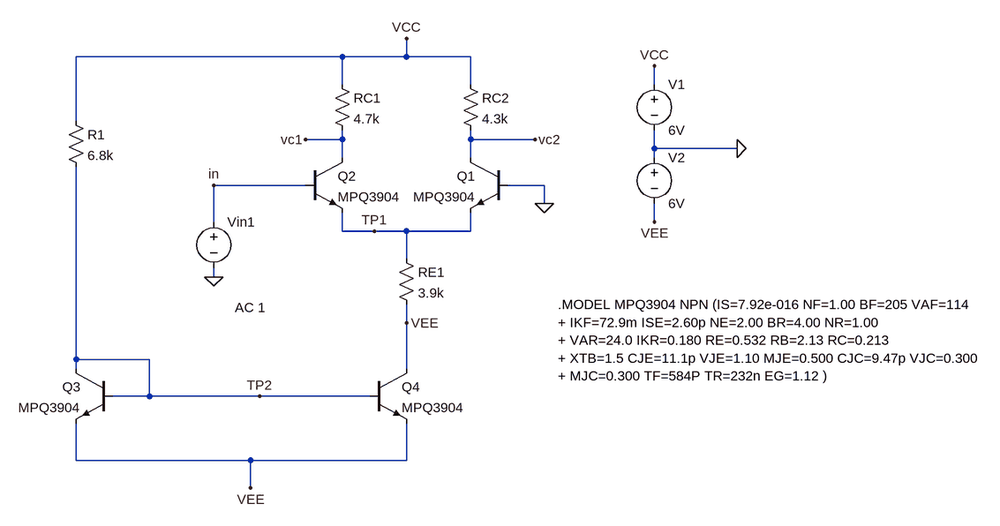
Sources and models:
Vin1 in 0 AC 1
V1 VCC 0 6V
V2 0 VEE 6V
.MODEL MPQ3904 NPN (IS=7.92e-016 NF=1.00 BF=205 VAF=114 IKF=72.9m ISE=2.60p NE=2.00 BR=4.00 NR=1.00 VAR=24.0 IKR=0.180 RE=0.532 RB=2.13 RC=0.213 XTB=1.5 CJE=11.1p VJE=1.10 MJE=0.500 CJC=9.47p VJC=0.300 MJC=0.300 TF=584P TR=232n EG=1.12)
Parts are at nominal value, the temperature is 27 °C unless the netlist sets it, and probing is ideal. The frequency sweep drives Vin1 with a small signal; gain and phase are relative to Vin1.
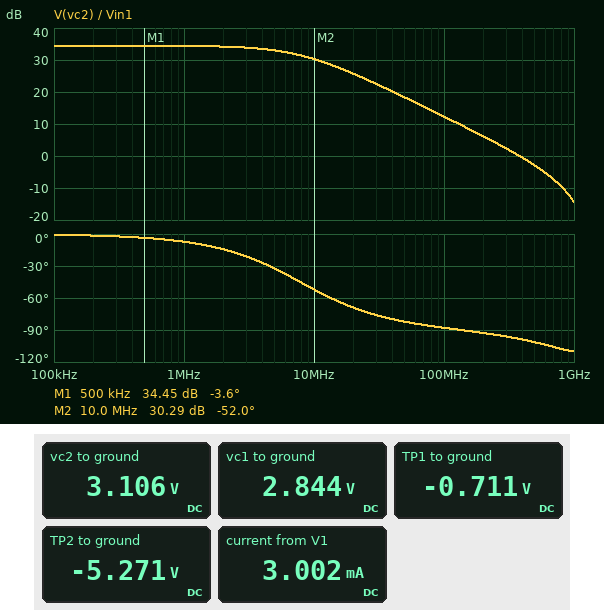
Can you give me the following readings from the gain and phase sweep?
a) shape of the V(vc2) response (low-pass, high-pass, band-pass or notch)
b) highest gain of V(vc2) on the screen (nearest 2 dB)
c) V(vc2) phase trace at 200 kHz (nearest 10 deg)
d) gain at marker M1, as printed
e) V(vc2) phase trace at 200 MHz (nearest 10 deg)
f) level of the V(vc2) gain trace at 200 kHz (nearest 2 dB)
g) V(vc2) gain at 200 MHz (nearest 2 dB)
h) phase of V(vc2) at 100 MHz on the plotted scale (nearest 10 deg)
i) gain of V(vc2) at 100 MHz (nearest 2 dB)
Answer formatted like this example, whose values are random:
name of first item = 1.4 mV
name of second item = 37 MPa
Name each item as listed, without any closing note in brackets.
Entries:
shape of the V(vc2) response = low-pass
highest gain of V(vc2) on the screen = 34 dB
V(vc2) phase trace at 200 kHz = 0 deg
gain at marker M1, as printed = 34.45 dB
V(vc2) phase trace at 200 MHz = -90 deg
level of the V(vc2) gain trace at 200 kHz = 34 dB
V(vc2) gain at 200 MHz = 6 dB
phase of V(vc2) at 100 MHz on the plotted scale = -90 deg
gain of V(vc2) at 100 MHz = 12 dB
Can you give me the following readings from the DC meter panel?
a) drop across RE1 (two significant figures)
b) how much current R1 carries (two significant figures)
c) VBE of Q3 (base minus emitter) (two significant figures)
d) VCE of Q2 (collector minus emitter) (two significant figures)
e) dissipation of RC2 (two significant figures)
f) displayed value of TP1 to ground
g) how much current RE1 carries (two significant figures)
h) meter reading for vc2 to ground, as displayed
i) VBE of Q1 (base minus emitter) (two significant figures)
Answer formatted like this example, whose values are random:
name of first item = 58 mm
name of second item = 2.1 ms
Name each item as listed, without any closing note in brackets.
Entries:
drop across RE1 = 5.3 V
how much current R1 carries = 1.7 mA
VBE of Q3 (base minus emitter) = 730 mV
VCE of Q2 (collector minus emitter) = 3.6 V
dissipation of RC2 = 1.9 mW
displayed value of TP1 to ground = -0.711 V
how much current RE1 carries = 1.4 mA
meter reading for vc2 to ground, as displayed = 3.106 V
VBE of Q1 (base minus emitter) = 710 mV
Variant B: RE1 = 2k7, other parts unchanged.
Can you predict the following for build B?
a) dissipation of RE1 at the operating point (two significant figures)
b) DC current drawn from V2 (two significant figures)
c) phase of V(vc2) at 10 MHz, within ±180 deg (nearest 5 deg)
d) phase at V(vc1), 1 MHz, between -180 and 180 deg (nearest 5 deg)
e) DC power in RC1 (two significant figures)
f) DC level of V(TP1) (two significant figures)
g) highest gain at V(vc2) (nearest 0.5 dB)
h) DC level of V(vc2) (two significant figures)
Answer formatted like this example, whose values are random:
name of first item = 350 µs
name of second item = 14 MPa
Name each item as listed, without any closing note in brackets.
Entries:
dissipation of RE1 at the operating point = 10 mW
DC current drawn from V2 = 3.6 mA
phase of V(vc2) at 10 MHz, within ±180 deg = -55 deg
phase at V(vc1), 1 MHz, between -180 and 180 deg = 170 deg
DC power in RC1 = 4.4 mW
DC level of V(TP1) = -720 mV
highest gain at V(vc2) = 37.5 dB
DC level of V(vc2) = 1.8 V
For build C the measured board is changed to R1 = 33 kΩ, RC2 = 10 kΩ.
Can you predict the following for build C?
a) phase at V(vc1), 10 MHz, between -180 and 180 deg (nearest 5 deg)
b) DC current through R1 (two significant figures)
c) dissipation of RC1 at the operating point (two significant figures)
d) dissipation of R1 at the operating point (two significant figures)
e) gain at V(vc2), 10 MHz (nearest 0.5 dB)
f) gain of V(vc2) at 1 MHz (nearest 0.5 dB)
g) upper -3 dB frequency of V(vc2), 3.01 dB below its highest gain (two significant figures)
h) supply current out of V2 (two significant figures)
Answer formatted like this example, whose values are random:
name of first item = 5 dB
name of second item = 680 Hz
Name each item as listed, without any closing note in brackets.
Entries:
phase at V(vc1), 10 MHz, between -180 and 180 deg = 125 deg
DC current through R1 = 340 µA
dissipation of RC1 at the operating point = 2.2 mW
dissipation of R1 at the operating point = 3.9 mW
gain at V(vc2), 10 MHz = 9.0 dB
gain of V(vc2) at 1 MHz = 28.0 dB
upper -3 dB frequency of V(vc2), 3.01 dB below its highest gain = 570 kHz
supply current out of V2 = 1.7 mA
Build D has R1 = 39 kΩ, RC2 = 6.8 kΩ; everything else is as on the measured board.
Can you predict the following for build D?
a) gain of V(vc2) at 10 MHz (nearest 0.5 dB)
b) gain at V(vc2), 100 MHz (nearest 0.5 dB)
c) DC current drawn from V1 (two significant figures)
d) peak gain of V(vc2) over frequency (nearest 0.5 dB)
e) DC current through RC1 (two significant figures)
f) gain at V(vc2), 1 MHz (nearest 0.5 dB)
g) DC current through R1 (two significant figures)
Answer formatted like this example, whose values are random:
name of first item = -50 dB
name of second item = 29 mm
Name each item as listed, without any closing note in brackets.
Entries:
gain of V(vc2) at 10 MHz = 30.0 dB
gain at V(vc2), 100 MHz = 10.5 dB
DC current drawn from V1 = 1.6 mA
peak gain of V(vc2) over frequency = 38.5 dB
DC current through RC1 = 680 µA
gain at V(vc2), 1 MHz = 38.0 dB
DC current through R1 = 290 µA
